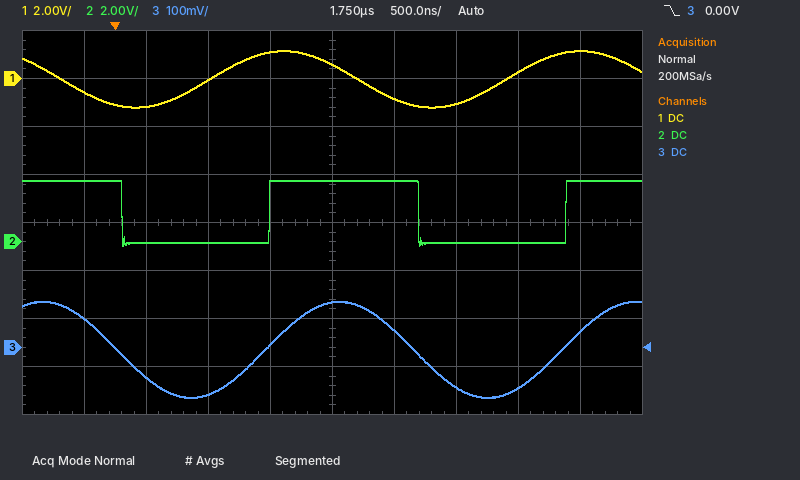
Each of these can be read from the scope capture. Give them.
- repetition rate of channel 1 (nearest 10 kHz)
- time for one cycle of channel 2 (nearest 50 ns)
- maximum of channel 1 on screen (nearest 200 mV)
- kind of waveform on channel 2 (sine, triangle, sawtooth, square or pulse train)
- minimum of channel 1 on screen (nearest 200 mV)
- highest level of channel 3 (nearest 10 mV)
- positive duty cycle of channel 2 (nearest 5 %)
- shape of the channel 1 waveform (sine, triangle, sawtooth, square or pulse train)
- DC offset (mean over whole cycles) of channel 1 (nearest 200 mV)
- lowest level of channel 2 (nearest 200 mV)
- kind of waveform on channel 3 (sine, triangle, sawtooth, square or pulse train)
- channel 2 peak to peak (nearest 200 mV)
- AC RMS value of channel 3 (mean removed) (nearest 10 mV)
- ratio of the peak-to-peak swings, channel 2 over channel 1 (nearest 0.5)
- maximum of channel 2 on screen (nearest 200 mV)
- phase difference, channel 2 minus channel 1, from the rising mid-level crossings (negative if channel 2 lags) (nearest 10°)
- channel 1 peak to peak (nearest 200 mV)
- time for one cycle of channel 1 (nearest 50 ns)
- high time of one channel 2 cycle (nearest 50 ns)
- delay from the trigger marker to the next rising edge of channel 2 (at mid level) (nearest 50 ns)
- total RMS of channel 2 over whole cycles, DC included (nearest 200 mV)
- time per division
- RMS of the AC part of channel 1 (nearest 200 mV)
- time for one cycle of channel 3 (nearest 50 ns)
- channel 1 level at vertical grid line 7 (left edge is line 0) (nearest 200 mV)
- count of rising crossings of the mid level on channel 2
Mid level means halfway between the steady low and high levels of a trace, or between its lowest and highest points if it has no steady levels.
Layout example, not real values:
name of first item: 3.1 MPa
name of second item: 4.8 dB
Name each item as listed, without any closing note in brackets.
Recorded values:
repetition rate of channel 1: 420 kHz
time for one cycle of channel 2: 2.40 µs
maximum of channel 1 on screen: 1.2 V
kind of waveform on channel 2: square
minimum of channel 1 on screen: -1.2 V
highest level of channel 3: 100 mV
positive duty cycle of channel 2: 50 %
shape of the channel 1 waveform: sine
DC offset (mean over whole cycles) of channel 1: 0.0 V
lowest level of channel 2: -200 mV
kind of waveform on channel 3: sine
channel 2 peak to peak: 2.8 V
AC RMS value of channel 3 (mean removed): 70 mV
ratio of the peak-to-peak swings, channel 2 over channel 1: 1.0
maximum of channel 2 on screen: 2.6 V
phase difference, channel 2 minus channel 1, from the rising mid-level crossings (negative if channel 2 lags): -70°
channel 1 peak to peak: 2.4 V
time for one cycle of channel 1: 2.40 µs
high time of one channel 2 cycle: 1.20 µs
delay from the trigger marker to the next rising edge of channel 2 (at mid level): 1.25 µs
total RMS of channel 2 over whole cycles, DC included: 1.8 V
time per division: 500 ns
RMS of the AC part of channel 1: 800 mV
time for one cycle of channel 3: 2.40 µs
channel 1 level at vertical grid line 7 (left edge is line 0): -1.0 V
count of rising crossings of the mid level on channel 2: 2
